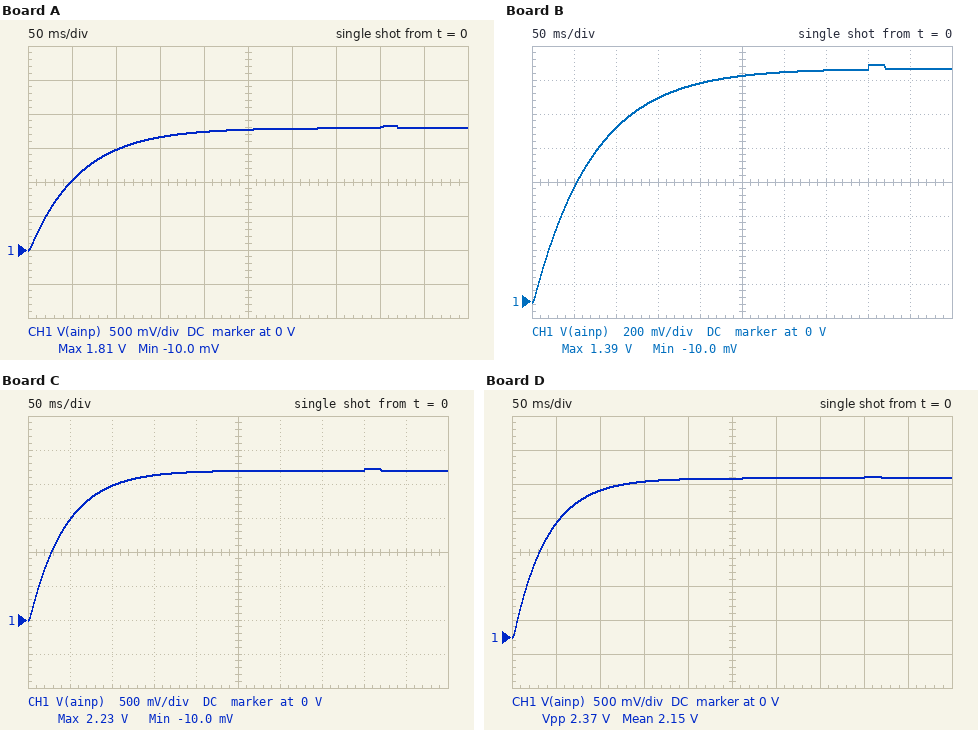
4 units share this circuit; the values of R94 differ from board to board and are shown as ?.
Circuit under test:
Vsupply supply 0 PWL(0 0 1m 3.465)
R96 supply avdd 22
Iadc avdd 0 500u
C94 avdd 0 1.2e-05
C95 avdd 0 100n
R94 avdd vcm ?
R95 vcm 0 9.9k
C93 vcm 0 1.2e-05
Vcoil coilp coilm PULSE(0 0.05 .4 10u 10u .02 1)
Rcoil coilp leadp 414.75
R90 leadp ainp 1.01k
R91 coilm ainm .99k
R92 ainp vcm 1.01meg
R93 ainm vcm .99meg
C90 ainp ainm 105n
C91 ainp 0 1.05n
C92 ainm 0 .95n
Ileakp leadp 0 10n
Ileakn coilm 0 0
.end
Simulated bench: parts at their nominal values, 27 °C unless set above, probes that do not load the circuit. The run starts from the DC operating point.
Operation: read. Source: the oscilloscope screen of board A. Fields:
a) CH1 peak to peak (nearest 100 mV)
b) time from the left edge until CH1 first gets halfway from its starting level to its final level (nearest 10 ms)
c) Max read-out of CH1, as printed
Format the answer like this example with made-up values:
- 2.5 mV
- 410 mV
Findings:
- 1.8 V
- 40 ms
- 1.81 V
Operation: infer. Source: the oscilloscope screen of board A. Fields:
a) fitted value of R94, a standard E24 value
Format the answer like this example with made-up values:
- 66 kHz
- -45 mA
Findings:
- 9.1 kΩ
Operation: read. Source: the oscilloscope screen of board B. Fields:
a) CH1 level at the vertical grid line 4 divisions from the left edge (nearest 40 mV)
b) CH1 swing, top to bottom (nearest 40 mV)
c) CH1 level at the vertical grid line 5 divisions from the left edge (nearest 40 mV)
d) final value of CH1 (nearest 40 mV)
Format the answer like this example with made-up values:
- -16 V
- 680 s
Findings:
- 1.28 V
- 1.40 V
- 1.32 V
- 1.36 V
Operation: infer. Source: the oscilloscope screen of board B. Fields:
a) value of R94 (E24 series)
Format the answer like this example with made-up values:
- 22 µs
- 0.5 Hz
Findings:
- 15 kΩ
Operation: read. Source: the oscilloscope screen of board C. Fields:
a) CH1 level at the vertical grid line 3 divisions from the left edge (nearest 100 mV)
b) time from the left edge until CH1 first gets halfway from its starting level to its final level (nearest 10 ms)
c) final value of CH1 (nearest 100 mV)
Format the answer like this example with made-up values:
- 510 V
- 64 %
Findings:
- 2.1 V
- 30 ms
- 2.2 V
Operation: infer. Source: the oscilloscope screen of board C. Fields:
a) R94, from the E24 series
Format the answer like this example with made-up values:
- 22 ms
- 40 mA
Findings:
- 5.6 kΩ
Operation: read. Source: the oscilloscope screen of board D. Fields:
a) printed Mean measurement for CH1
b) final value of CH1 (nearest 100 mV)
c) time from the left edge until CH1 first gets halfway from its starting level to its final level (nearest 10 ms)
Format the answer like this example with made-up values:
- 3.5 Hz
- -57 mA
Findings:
- 2.15 V
- 2.3 V
- 30 ms
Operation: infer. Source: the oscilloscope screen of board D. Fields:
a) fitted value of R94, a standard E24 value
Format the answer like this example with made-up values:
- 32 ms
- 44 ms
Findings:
- 4.7 kΩ
